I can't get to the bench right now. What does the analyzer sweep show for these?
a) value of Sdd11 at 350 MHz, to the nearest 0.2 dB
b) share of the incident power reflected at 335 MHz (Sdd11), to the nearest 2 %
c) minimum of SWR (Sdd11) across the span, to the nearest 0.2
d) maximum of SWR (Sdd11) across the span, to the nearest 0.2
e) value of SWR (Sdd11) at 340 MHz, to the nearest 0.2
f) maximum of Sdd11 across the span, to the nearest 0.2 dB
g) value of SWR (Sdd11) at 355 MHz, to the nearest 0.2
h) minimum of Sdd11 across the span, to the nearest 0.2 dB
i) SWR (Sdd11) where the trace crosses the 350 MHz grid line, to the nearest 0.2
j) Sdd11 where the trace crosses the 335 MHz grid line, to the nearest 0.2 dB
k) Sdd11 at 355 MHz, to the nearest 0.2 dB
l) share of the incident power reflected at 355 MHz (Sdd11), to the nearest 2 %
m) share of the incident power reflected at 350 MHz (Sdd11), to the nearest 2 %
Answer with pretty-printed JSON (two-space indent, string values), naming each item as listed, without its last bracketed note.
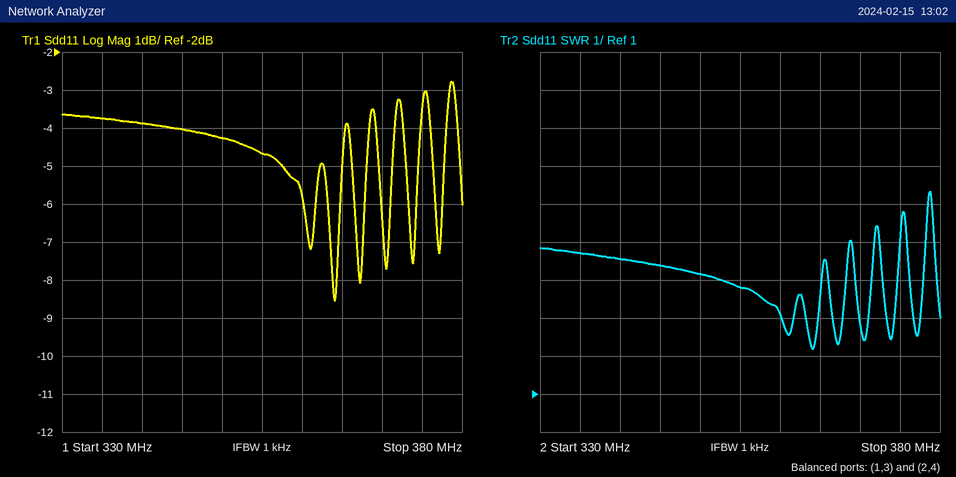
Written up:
{
  "value of Sdd11 at 350 MHz, to the nearest 0.2 dB": "-4.2 dB",
  "share of the incident power reflected at 335 MHz (Sdd11), to the nearest 2 %": "42 %",
  "minimum of SWR (Sdd11) across the span, to the nearest 0.2": "2.2",
  "maximum of SWR (Sdd11) across the span, to the nearest 0.2": "6.4",
  "value of SWR (Sdd11) at 340 MHz, to the nearest 0.2": "4.6",
  "maximum of Sdd11 across the span, to the nearest 0.2 dB": "-2.8 dB",
  "value of SWR (Sdd11) at 355 MHz, to the nearest 0.2": "3.8",
  "minimum of Sdd11 across the span, to the nearest 0.2 dB": "-8.6 dB",
  "SWR (Sdd11) where the trace crosses the 350 MHz grid line, to the nearest 0.2": "4.2",
  "Sdd11 where the trace crosses the 335 MHz grid line, to the nearest 0.2 dB": "-3.8 dB",
  "Sdd11 at 355 MHz, to the nearest 0.2 dB": "-4.6 dB",
  "share of the incident power reflected at 355 MHz (Sdd11), to the nearest 2 %": "34 %",
  "share of the incident power reflected at 350 MHz (Sdd11), to the nearest 2 %": "38 %"
}
